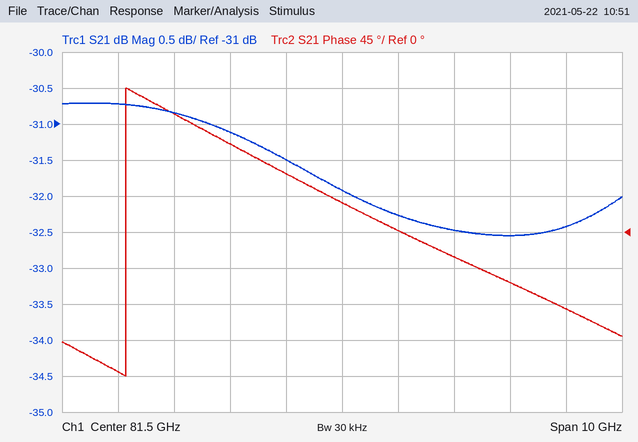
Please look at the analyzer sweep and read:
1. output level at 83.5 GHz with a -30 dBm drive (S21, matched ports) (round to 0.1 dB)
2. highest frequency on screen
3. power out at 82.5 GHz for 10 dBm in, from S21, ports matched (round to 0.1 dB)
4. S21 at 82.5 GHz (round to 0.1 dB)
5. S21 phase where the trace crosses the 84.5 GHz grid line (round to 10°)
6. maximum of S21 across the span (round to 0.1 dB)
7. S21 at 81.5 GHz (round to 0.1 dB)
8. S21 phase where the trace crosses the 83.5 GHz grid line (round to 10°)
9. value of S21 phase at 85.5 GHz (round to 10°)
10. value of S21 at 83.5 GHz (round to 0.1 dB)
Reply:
-62.5 dBm
86.5 GHz
-22.3 dBm
-32.3 dB
-60°
-30.7 dB
-31.9 dB
-30°
-100°
-32.5 dB
